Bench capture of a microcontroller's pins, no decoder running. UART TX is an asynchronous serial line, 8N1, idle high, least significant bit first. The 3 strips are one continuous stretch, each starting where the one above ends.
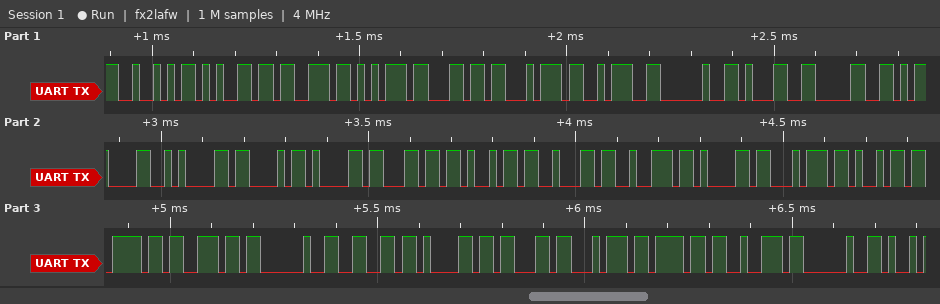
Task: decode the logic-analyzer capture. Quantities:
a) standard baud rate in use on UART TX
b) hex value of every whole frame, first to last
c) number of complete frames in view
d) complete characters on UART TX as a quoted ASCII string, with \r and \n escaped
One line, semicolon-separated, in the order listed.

57600 baud; 52 65 73 75 6C 74 3A 20 31 30 0D 0A 43 61 6C 69 62 72 61 74 69 6F 6E 20 66 61 63 74 6F 72 20; 31; "Result: 10\r\nCalibration factor "
